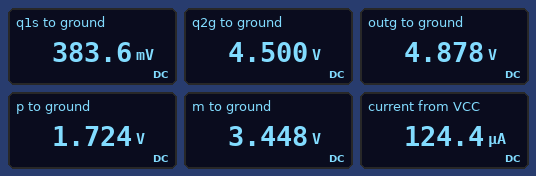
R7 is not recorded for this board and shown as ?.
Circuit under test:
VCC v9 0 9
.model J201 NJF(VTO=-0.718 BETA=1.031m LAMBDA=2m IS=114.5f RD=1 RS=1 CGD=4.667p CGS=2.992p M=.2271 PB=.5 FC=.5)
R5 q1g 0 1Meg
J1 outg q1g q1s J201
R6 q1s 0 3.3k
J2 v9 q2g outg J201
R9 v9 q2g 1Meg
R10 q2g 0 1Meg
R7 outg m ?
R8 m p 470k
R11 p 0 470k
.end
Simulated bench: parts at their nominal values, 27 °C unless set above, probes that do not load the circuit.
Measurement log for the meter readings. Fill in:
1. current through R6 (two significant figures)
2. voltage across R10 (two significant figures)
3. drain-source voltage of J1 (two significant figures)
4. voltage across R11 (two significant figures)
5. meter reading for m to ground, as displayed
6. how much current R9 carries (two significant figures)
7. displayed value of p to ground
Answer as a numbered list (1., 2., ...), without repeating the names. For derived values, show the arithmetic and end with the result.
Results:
1. (383.6 mV) / 3.3 kΩ = 120 µA
2. 4.5 V = 4.5 V
3. 4.878 V - 383.6 mV = 4.5 V
4. 1.724 V = 1.7 V
5. 3.448 V
6. (9 V - 4.5 V) / 1 MΩ = 4.5 µA
7. 1.724 V
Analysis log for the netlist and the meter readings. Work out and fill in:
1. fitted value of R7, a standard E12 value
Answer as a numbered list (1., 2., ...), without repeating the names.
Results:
1. 390 kΩ
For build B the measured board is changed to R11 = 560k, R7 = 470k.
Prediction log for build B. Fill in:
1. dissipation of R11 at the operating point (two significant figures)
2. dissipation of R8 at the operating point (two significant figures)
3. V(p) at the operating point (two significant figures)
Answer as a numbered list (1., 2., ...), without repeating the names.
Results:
1. 5.9 µW
2. 5.0 µW
3. 1.8 V
